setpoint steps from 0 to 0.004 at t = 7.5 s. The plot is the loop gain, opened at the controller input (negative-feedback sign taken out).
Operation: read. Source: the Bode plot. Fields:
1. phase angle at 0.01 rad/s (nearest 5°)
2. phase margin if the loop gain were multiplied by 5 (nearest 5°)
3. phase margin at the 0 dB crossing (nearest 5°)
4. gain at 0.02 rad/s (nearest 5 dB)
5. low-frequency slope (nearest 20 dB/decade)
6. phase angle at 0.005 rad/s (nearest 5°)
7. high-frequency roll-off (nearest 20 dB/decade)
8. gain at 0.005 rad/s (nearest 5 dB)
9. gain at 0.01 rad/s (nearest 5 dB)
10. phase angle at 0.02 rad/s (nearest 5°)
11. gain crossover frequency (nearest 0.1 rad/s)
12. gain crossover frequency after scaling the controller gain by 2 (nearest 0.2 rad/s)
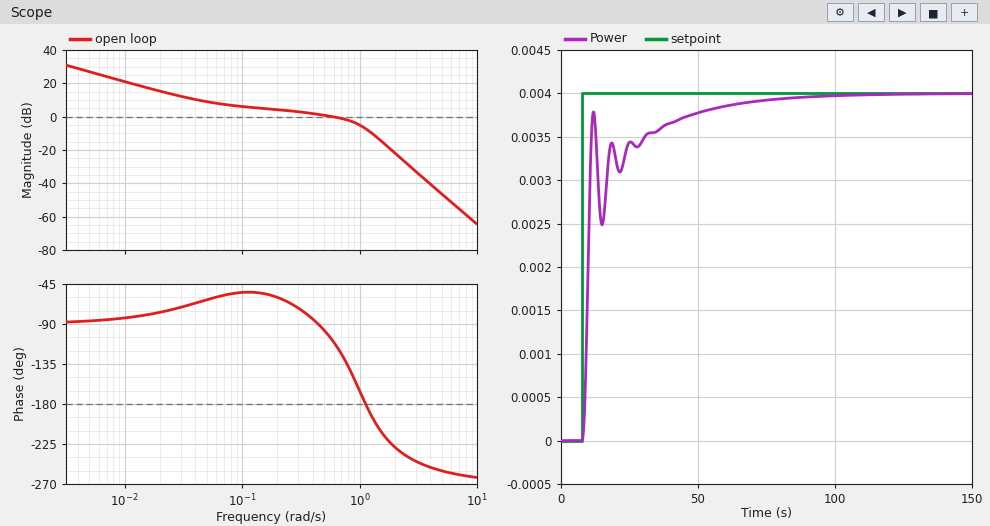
-85°
-30°
70°
15 dB
-20 dB/decade
-85°
-60 dB/decade
25 dB
20 dB
-75°
0.6 rad/s
1.0 rad/s
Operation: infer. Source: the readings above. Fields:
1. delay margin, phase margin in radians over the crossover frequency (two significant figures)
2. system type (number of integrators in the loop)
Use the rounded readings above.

2.0 s
1
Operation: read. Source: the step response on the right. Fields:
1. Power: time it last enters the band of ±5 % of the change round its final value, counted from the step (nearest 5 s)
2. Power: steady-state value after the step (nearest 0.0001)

45 s
0.0040
